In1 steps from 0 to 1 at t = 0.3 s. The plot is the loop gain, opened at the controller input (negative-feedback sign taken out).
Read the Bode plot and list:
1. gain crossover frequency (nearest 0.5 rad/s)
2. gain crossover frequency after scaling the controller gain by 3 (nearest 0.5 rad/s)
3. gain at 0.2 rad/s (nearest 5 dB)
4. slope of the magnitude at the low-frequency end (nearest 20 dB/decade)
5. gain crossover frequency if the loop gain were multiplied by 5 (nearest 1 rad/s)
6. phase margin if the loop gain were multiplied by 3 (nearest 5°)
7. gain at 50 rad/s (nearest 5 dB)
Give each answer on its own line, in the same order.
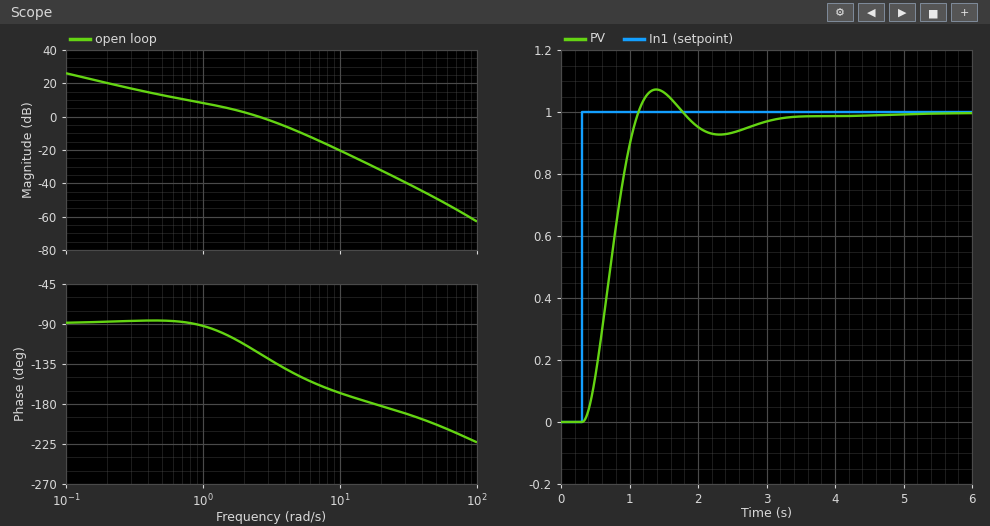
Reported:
2.5 rad/s
5.0 rad/s
20 dB
-20 dB/decade
7 rad/s
30°
-50 dB
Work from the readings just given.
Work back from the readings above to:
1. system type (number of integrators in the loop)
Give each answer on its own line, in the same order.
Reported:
1
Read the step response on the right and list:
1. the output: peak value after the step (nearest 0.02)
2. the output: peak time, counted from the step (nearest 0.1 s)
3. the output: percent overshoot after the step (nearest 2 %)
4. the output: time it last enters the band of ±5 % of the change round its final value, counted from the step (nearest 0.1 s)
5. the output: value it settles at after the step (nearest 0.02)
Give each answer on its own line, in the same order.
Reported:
1.08
1.1 s
8 %
2.4 s
1.00
